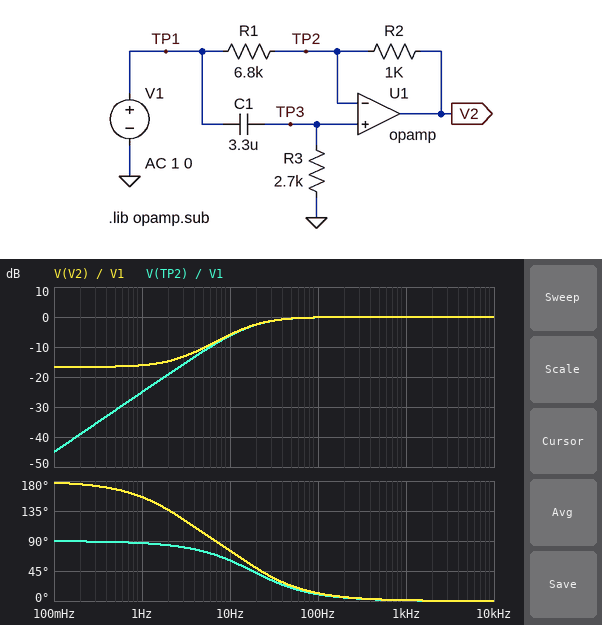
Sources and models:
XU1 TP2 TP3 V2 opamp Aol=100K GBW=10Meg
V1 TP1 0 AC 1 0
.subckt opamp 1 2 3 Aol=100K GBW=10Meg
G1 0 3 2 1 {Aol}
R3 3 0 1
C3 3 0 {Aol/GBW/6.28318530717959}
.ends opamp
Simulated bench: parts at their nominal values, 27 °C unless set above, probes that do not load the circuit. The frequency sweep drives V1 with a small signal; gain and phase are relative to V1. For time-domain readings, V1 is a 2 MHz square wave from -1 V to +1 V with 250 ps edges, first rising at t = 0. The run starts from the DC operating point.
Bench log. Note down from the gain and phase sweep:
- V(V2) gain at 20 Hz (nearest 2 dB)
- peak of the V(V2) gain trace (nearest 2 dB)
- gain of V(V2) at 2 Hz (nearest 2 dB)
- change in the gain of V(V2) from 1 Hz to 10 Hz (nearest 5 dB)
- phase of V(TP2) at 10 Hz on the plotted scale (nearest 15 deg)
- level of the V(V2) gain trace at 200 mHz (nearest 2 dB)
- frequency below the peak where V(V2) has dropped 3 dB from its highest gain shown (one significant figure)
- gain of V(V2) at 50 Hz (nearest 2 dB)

-2 dB
0 dB
-14 dB
10 dB
60 deg
-16 dB
20 Hz
0 dB
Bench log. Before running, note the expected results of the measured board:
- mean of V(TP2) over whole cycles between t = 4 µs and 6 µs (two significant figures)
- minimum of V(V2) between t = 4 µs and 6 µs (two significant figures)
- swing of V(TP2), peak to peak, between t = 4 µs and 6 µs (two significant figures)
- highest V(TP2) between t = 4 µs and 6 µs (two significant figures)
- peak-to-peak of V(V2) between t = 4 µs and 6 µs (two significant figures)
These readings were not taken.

1.0 V
150 mV
2.0 V
2.0 V
2.0 V
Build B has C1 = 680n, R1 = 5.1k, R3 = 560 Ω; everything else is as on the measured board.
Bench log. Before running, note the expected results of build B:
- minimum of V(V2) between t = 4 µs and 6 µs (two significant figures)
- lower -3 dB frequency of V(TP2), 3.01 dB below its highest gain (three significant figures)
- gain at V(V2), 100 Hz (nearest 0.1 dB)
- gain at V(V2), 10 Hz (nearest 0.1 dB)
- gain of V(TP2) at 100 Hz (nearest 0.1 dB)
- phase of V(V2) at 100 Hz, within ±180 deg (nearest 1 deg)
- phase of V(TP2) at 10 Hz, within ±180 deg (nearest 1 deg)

180 mV
418 Hz
-10.4 dB
-14.1 dB
-12.7 dB
116 deg
89 deg
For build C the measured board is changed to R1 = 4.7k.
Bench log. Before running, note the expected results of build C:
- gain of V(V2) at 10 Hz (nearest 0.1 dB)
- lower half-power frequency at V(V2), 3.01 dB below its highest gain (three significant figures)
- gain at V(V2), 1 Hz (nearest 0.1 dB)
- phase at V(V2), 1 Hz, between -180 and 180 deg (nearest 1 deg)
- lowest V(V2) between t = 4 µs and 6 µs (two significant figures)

-5.6 dB
17.0 Hz
-13.2 dB
162 deg
210 mV
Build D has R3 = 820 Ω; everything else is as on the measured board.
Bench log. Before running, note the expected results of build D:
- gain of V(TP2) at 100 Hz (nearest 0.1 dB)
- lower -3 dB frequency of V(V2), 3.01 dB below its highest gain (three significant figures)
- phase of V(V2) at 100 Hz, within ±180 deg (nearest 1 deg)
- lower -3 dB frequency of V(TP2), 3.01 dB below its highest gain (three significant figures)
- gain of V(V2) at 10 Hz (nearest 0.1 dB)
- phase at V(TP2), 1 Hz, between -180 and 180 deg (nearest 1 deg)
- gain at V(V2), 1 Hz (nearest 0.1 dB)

-1.3 dB
57.5 Hz
35 deg
58.8 Hz
-13.1 dB
89 deg
-16.6 dB
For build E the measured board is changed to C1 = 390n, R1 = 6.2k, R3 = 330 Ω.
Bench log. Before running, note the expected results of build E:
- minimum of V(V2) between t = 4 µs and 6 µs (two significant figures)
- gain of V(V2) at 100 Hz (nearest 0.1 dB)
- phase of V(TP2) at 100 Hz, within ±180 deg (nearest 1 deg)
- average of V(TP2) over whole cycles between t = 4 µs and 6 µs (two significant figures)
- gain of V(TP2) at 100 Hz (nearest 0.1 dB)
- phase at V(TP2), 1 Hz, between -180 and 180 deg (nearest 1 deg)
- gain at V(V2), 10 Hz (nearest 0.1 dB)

110 mV
-14.9 dB
85 deg
960 mV
-21.9 dB
90 deg
-15.8 dB
